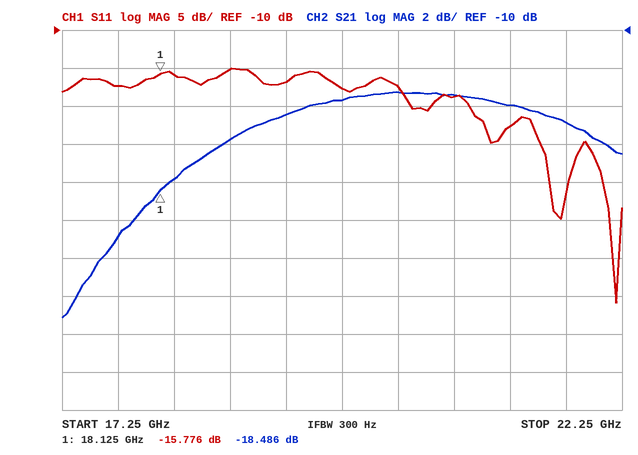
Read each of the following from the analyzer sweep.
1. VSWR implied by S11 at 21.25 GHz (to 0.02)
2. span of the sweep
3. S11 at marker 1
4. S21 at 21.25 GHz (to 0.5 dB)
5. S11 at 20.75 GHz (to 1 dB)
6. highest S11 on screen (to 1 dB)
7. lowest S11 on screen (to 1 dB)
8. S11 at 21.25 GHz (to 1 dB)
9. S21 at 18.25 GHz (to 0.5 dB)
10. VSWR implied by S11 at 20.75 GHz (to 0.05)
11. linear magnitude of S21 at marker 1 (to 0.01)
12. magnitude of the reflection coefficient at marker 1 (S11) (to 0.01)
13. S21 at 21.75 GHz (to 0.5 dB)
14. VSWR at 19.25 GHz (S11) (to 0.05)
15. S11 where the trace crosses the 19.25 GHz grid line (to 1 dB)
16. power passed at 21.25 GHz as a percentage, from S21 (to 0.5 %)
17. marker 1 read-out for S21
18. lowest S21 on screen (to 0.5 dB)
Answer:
1.16
5 GHz
-15.776 dB
-14.0 dB
-19 dB
-15 dB
-46 dB
-23 dB
-18.0 dB
1.25
0.12
0.16
-15.0 dB
1.35
-17 dB
4.0 %
-18.486 dB
-25.0 dB
